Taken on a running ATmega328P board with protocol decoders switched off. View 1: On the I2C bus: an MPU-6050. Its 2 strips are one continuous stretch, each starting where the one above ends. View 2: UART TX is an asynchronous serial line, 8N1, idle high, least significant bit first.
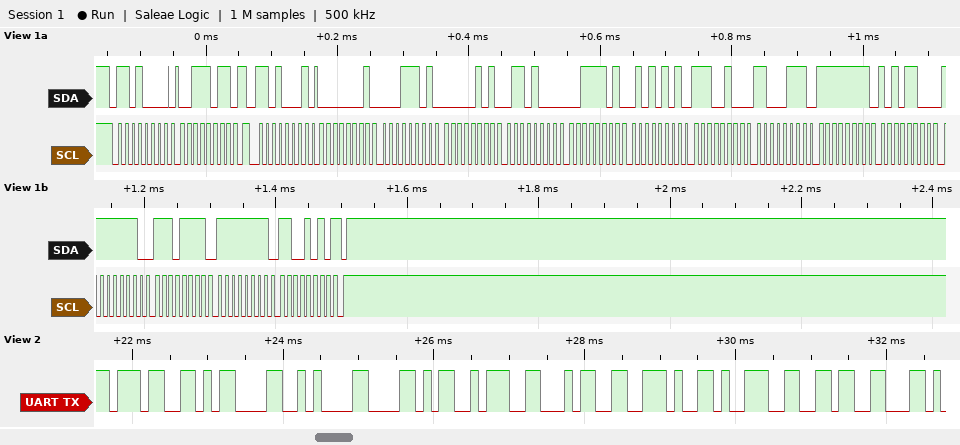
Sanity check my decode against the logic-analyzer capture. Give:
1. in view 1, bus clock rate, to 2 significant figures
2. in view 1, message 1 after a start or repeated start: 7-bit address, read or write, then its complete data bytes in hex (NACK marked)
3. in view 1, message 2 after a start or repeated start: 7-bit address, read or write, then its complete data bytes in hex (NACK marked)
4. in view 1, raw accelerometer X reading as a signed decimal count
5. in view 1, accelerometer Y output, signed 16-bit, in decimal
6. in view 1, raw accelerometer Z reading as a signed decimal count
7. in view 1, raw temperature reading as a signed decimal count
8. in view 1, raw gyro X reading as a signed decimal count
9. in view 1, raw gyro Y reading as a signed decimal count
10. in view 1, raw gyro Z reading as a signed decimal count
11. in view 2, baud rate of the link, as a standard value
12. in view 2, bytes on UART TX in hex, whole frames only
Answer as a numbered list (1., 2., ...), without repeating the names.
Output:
1. 100 kHz
2. 0x68 write: 3B
3. 0x68 read: 01 1D 05 68 3D 55 E4 C7 FF AC FE EF FF CA NACK
4. 285
5. 1384
6. 15701
7. -6969
8. -84
9. -273
10. -54
11. 9600 baud
12. 37 0D 0A 58 3A 34 2E 39 36
